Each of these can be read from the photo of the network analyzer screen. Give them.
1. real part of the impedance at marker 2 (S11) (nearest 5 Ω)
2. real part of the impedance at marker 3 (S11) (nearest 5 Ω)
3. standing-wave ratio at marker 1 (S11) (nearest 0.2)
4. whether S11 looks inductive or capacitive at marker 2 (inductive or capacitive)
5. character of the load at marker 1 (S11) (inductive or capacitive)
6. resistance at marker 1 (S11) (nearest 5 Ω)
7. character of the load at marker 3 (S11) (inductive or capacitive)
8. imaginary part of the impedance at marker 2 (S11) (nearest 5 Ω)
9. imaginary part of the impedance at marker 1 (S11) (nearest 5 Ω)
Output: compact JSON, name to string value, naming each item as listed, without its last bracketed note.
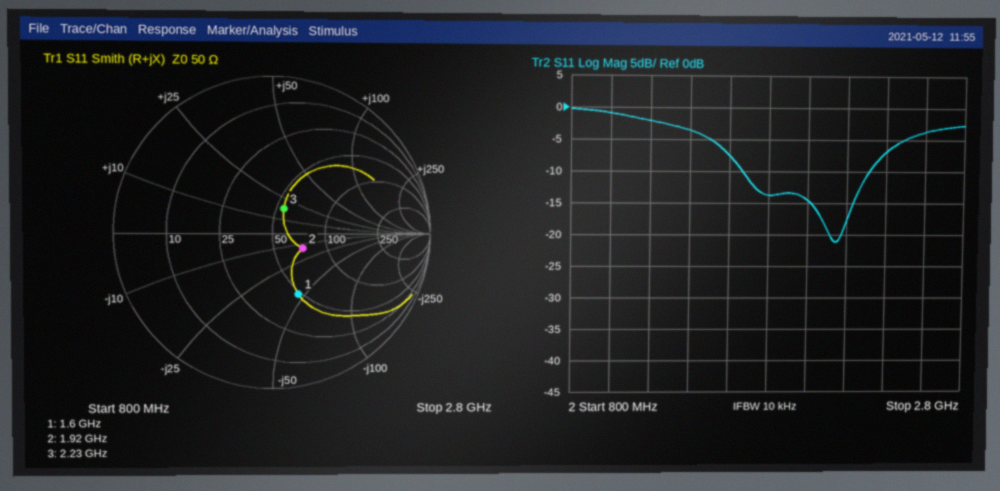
{"real part of the impedance at marker 2 (S11)": "70 Ω", "real part of the impedance at marker 3 (S11)": "55 Ω", "standing-wave ratio at marker 1 (S11)": "2.4", "whether S11 looks inductive or capacitive at marker 2": "capacitive", "character of the load at marker 1 (S11)": "capacitive", "resistance at marker 1 (S11)": "50 Ω", "character of the load at marker 3 (S11)": "inductive", "imaginary part of the impedance at marker 2 (S11)": "-15 Ω", "imaginary part of the impedance at marker 1 (S11)": "-45 Ω"}
